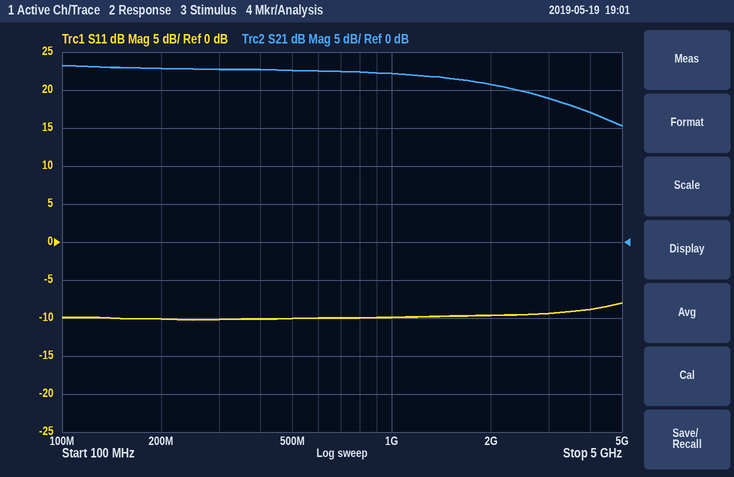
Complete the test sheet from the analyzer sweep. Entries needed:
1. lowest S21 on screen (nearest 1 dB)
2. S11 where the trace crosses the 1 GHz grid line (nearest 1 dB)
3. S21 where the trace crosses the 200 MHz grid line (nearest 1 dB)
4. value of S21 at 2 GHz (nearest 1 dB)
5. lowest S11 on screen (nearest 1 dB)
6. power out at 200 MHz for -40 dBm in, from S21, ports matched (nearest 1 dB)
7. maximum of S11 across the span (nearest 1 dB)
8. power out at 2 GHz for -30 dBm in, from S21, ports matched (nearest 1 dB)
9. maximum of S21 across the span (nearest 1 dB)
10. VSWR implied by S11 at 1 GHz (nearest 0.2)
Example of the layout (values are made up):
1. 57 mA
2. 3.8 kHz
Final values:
1. 15 dB
2. -10 dB
3. 23 dB
4. 21 dB
5. -10 dB
6. -17 dBm
7. -8 dB
8. -9 dBm
9. 23 dB
10. 2.0
